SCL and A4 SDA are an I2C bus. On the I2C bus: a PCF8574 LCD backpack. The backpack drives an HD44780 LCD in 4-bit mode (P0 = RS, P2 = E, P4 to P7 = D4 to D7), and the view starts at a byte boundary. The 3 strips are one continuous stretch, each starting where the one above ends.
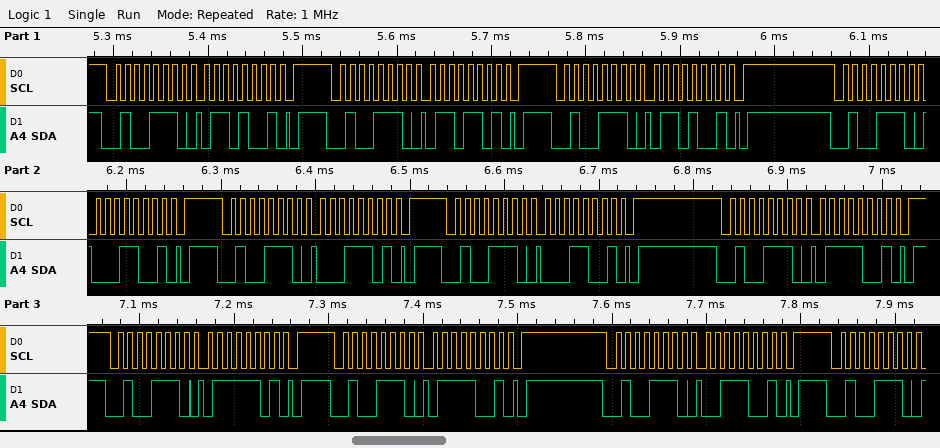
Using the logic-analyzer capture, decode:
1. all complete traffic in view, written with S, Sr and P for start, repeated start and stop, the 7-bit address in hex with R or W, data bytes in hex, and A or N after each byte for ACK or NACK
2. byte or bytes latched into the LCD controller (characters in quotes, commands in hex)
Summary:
S 27W A 69 A P S 27W A 6D A P S 27W A 69 A P S 27W A 19 A P S 27W A 1D A P S 27W A 19 A P S 27W A 79 A P S 27W A 7D A P S 27W A 79 A P S 27W A 39 A P S 27W A
'a'
